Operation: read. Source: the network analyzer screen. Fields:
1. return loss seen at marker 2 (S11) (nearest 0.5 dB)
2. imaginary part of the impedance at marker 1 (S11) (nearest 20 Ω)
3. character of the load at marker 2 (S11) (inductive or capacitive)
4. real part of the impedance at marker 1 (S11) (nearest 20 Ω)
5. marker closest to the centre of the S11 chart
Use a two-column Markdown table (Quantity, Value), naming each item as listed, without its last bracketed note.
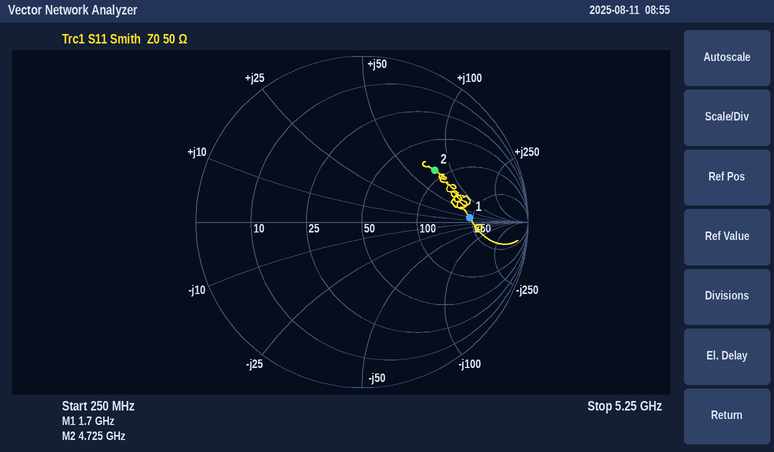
| Quantity | Value |
|---|---|
| return loss seen at marker 2 (S11) | 5.5 dB |
| imaginary part of the impedance at marker 1 (S11) | +20 Ω |
| character of the load at marker 2 (S11) | inductive |
| real part of the impedance at marker 1 (S11) | 240 Ω |
| marker closest to the centre of the S11 chart | marker 2 |
